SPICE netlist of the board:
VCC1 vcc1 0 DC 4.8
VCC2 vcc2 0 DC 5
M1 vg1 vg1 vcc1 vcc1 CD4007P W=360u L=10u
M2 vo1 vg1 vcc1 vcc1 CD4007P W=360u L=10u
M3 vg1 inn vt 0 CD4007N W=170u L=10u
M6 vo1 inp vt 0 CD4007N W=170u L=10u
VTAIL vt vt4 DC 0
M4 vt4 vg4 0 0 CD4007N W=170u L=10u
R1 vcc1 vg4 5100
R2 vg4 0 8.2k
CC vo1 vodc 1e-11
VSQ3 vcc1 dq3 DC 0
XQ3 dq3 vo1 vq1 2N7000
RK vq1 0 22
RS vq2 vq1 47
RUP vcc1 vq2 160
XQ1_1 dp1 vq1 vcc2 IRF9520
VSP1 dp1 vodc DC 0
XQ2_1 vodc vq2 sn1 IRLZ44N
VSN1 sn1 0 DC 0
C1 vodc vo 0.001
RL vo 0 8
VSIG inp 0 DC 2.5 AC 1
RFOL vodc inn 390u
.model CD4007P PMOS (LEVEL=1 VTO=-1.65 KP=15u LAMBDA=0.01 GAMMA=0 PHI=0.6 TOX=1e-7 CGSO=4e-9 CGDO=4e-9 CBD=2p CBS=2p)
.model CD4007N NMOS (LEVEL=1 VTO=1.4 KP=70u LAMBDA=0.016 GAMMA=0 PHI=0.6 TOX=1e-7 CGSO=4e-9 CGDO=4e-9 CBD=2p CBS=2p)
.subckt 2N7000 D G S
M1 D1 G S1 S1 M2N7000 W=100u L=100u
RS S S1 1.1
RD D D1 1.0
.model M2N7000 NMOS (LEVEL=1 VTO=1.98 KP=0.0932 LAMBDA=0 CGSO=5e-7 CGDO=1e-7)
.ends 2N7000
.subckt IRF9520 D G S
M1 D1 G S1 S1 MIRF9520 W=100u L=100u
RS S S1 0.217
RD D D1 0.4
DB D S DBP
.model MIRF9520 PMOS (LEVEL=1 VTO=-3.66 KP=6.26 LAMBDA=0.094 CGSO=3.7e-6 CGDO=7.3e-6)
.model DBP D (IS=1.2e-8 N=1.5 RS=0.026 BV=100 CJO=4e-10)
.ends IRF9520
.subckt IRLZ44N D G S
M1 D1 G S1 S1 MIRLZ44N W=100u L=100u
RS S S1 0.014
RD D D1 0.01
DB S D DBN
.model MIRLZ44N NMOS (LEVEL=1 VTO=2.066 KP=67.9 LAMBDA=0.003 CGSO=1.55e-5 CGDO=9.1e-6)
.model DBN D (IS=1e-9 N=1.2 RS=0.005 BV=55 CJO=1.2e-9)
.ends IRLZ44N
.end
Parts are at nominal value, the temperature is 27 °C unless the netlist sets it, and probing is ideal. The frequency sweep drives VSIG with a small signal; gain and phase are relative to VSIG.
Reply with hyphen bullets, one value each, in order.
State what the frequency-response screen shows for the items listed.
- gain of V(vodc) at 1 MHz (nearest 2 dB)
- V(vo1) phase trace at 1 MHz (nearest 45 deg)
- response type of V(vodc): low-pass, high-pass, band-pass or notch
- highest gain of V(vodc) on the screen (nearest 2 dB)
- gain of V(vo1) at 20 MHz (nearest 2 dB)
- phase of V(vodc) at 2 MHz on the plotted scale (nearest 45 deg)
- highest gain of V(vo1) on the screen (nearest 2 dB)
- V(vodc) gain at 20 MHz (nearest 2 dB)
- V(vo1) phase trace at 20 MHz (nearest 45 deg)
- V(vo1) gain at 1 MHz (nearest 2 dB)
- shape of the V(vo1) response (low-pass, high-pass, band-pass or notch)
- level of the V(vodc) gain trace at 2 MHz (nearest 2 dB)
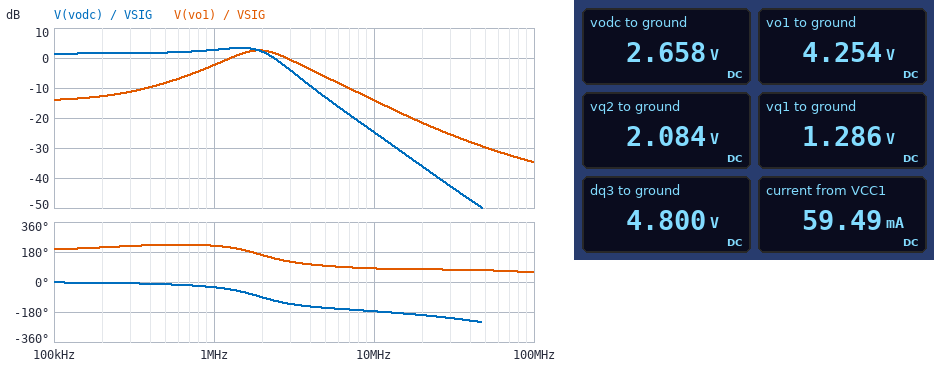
- 2 dB
- 225 deg
- low-pass
- 4 dB
- -22 dB
- -90 deg
- 2 dB
- -36 dB
- 90 deg
- -2 dB
- band-pass
- 2 dB
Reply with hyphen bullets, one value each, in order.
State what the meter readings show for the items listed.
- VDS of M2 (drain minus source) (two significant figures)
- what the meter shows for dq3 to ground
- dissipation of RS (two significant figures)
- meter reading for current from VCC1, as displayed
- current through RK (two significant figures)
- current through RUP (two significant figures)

- -550 mV
- 4.800 V
- 14 mW
- 59.49 mA
- 58 mA
- 17 mA
